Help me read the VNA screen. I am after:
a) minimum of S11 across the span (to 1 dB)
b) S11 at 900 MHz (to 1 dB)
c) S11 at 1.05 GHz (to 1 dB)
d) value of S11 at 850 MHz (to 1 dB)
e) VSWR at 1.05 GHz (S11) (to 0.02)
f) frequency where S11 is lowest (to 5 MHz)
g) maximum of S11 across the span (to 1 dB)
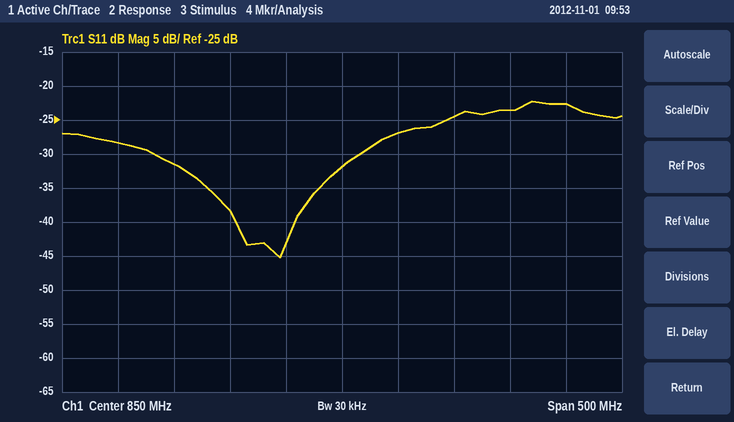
-45 dB
-27 dB
-23 dB
-32 dB
1.16
795 MHz
-22 dB
